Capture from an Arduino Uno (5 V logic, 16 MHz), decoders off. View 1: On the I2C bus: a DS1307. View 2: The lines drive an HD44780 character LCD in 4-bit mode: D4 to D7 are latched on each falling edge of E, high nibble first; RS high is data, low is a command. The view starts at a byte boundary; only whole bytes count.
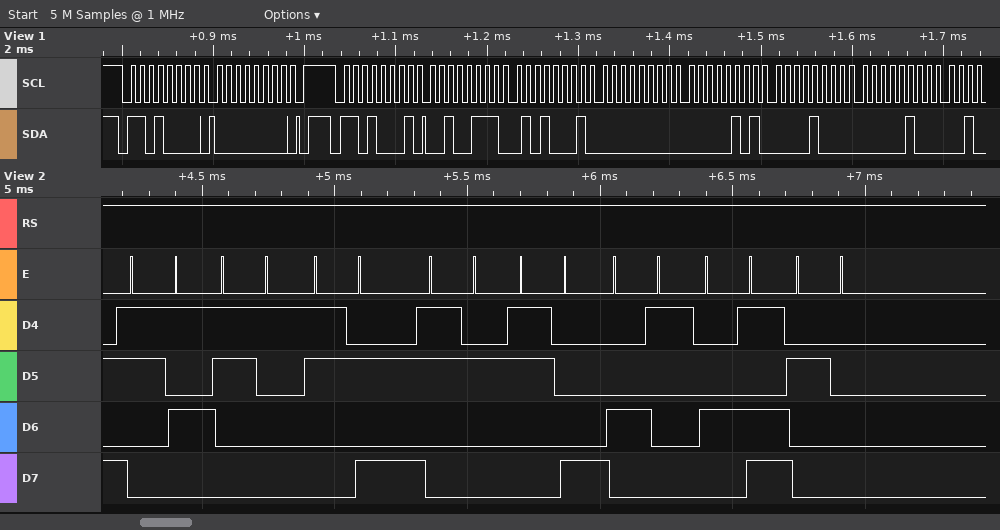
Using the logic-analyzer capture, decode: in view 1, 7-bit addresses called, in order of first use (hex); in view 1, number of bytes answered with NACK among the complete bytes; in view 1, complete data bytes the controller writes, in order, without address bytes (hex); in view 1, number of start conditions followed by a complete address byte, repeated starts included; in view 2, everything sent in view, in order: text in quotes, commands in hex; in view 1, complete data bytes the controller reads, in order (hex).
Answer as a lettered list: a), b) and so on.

a) 0x68
b) 0
c) 00
d) 2
e) "51:28AM "
f) 27 51 00 05 08 04
